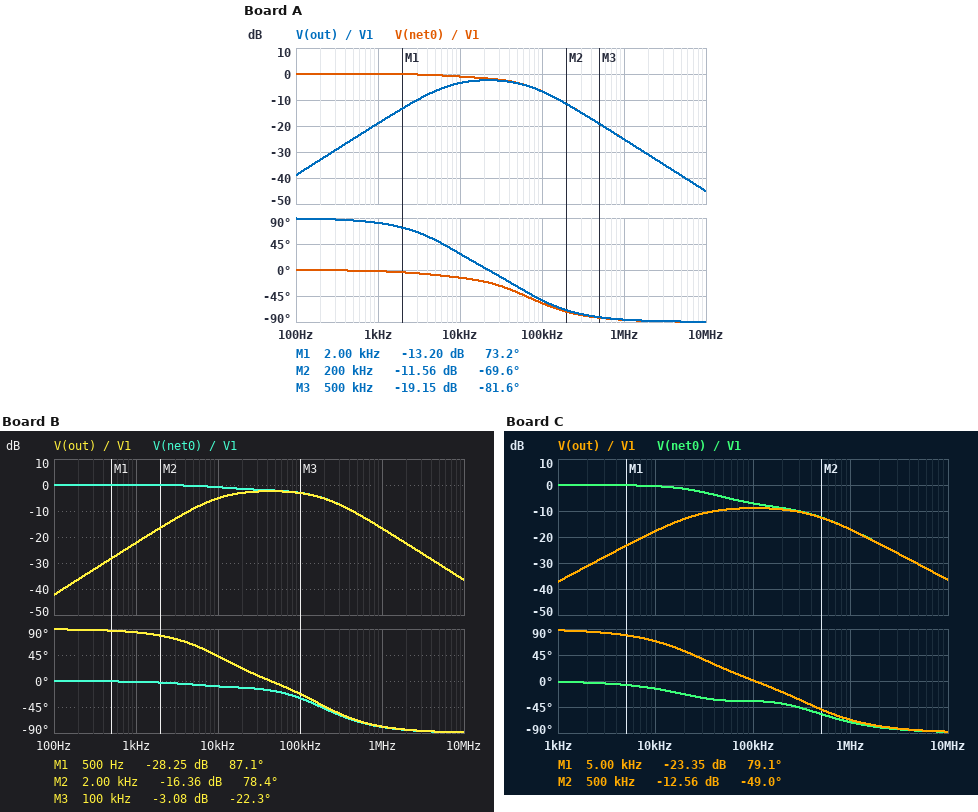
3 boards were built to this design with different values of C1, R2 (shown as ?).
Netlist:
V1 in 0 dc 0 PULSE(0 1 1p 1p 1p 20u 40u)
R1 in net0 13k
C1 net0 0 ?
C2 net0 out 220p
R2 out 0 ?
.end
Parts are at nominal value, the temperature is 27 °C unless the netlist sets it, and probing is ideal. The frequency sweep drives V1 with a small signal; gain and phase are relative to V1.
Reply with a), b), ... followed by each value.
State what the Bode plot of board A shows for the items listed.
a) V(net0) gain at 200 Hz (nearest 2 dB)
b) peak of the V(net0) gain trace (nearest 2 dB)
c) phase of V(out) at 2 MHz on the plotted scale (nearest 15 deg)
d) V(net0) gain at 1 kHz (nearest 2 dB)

a) 0 dB
b) 0 dB
c) -90 deg
d) 0 dB
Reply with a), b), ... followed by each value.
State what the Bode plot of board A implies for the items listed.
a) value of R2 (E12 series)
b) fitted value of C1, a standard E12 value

a) 82 kΩ
b) 220 pF
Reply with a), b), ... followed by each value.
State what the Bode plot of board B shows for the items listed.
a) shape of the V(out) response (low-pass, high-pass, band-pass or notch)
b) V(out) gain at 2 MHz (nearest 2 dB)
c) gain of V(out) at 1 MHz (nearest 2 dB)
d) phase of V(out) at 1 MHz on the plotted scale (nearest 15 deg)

a) band-pass
b) -22 dB
c) -16 dB
d) -75 deg
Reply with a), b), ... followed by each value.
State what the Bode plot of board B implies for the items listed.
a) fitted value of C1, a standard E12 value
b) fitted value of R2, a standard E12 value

a) 82 pF
b) 56 kΩ
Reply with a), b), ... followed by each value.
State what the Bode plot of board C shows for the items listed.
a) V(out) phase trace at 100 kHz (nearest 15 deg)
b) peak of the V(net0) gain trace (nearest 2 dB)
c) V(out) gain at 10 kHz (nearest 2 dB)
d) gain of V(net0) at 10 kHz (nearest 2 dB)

a) 0 deg
b) 0 dB
c) -18 dB
d) 0 dB
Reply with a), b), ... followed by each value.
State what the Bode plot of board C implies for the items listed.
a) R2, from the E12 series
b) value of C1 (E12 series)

a) 10 kΩ
b) 82 pF
